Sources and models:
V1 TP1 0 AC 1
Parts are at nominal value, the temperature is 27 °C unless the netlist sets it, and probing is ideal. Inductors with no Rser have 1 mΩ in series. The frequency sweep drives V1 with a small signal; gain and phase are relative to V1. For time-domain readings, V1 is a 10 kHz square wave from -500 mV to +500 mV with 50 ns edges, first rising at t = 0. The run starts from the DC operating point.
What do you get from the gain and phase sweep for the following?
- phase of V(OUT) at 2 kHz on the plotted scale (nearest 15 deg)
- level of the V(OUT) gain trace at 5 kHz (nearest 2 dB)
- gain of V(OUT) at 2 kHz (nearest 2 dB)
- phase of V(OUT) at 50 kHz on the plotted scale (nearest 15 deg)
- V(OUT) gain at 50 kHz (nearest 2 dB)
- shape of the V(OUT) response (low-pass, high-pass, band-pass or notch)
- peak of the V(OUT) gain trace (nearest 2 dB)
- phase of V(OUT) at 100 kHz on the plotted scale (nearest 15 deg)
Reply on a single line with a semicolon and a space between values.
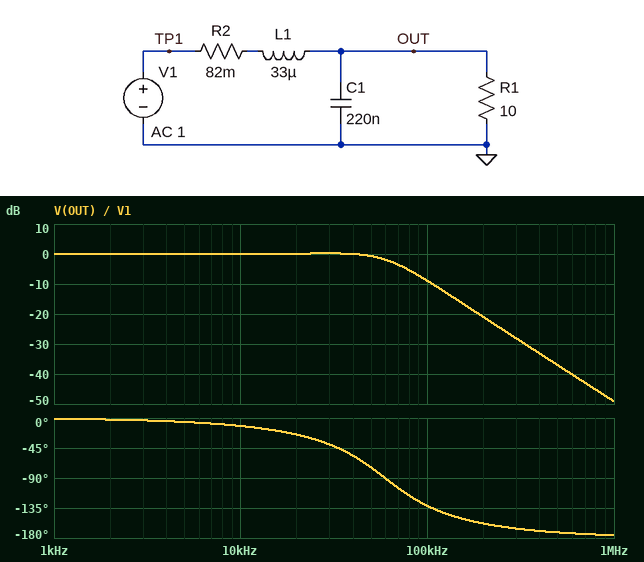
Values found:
0 deg; 0 dB; 0 dB; -75 deg; 0 dB; low-pass; 0 dB; -135 deg
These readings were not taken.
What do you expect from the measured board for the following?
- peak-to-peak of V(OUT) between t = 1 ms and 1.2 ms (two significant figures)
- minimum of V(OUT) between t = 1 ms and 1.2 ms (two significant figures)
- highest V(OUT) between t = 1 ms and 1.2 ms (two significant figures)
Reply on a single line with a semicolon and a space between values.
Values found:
1.2 V; -580 mV; 580 mV
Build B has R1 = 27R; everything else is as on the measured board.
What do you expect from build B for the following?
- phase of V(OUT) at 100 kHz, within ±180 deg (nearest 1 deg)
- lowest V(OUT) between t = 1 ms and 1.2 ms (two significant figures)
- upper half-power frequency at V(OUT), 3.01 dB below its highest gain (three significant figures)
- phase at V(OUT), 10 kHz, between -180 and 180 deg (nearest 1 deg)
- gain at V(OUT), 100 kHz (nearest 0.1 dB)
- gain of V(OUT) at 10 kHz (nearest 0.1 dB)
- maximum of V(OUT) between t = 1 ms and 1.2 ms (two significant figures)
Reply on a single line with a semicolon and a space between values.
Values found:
-157 deg; -970 mV; 68.5 kHz; -5 deg; -6.1 dB; 0.2 dB; 970 mV
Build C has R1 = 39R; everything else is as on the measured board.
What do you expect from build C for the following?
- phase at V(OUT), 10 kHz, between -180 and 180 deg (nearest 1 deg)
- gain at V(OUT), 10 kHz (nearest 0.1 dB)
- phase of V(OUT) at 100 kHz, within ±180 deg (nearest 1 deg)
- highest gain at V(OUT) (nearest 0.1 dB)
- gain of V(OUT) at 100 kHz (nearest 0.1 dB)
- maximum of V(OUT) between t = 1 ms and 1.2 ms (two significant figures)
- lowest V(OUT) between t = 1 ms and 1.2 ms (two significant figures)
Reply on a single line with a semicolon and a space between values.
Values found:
-3 deg; 0.2 dB; -164 deg; 10.0 dB; -5.8 dB; 1.1 V; -1.1 V
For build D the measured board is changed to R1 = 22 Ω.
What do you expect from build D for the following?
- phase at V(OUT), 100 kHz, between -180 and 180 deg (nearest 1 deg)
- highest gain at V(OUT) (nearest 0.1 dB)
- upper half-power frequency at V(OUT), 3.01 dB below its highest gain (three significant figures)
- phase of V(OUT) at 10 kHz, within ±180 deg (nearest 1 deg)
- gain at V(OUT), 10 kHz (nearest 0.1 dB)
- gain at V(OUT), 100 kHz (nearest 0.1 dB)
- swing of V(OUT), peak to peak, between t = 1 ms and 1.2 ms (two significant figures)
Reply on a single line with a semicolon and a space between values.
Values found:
-153 deg; 5.3 dB; 69.6 kHz; -6 deg; 0.2 dB; -6.4 dB; 1.8 V
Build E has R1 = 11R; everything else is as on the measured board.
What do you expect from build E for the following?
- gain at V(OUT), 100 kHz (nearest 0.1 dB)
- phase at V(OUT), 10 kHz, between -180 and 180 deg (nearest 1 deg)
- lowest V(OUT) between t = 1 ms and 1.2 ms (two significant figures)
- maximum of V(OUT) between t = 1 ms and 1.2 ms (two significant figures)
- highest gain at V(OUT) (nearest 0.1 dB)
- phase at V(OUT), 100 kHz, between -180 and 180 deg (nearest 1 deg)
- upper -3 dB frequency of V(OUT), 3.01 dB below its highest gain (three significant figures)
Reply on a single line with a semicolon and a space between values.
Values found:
-8.5 dB; -11 deg; -620 mV; 620 mV; 0.6 dB; -134 deg; 67.7 kHz
